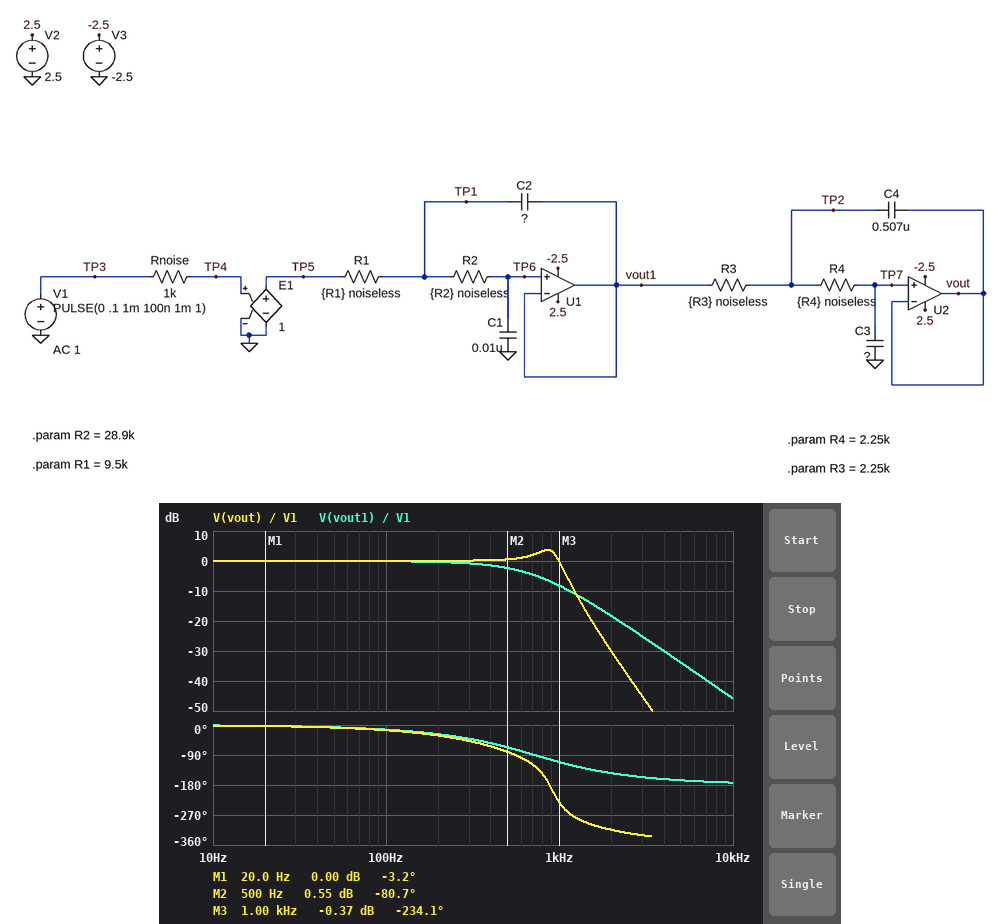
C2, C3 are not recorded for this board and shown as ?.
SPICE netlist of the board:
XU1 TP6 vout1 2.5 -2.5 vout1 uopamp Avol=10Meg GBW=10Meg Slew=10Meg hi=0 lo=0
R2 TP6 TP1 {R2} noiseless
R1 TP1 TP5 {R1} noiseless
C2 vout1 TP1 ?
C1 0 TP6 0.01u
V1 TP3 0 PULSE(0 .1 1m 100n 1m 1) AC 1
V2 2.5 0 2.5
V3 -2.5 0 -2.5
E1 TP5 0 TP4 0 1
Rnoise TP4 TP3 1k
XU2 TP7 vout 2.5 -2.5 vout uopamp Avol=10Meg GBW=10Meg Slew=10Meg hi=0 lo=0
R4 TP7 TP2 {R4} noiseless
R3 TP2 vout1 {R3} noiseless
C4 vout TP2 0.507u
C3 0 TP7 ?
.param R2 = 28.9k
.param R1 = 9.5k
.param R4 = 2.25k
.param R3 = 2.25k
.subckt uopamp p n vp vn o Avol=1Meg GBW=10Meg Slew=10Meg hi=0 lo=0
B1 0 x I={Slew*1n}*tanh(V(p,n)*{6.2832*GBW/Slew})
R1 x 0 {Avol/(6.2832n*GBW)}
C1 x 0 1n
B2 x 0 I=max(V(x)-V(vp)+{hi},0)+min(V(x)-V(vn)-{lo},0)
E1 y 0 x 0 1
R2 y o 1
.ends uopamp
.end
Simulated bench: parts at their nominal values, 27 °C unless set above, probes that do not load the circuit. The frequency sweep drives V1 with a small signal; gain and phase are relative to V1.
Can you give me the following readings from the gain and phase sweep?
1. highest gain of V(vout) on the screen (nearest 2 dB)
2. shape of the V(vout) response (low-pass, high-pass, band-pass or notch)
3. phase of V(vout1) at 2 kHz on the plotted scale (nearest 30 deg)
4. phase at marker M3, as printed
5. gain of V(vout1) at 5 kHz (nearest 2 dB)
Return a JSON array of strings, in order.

["4 dB", "low-pass", "-150 deg", "-234.1 deg", "-34 dB"]
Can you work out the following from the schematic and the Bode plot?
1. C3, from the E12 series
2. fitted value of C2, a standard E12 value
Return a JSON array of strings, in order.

["12 nF", "18 nF"]
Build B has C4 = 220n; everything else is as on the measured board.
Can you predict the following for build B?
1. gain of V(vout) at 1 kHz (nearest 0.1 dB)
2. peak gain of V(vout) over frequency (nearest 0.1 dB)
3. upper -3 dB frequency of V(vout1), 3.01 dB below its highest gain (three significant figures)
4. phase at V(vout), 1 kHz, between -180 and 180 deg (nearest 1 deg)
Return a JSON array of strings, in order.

["-3.6 dB", "0 dB", "565 Hz", "-147 deg"]
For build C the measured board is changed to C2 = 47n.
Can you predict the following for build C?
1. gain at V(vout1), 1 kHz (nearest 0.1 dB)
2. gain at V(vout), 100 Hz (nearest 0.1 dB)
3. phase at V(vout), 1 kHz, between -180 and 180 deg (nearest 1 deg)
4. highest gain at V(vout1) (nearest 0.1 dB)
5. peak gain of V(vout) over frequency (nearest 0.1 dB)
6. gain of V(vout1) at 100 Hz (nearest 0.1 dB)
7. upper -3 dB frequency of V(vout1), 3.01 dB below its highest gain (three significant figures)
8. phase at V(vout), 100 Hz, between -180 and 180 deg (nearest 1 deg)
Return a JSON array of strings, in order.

["-13.5 dB", "0.3 dB", "88 deg", "0.9 dB", "2.0 dB", "0.2 dB", "511 Hz", "-16 deg"]
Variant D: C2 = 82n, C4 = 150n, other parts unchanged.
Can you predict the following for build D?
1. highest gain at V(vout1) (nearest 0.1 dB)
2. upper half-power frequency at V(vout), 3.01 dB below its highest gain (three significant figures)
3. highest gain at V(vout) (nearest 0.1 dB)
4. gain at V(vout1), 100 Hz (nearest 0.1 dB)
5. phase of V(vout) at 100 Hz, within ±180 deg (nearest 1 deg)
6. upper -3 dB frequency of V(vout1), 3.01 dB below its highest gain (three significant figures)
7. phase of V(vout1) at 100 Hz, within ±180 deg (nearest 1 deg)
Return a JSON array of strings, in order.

["2.6 dB", "404 Hz", "2.8 dB", "0.5 dB", "-17 deg", "399 Hz", "-15 deg"]
